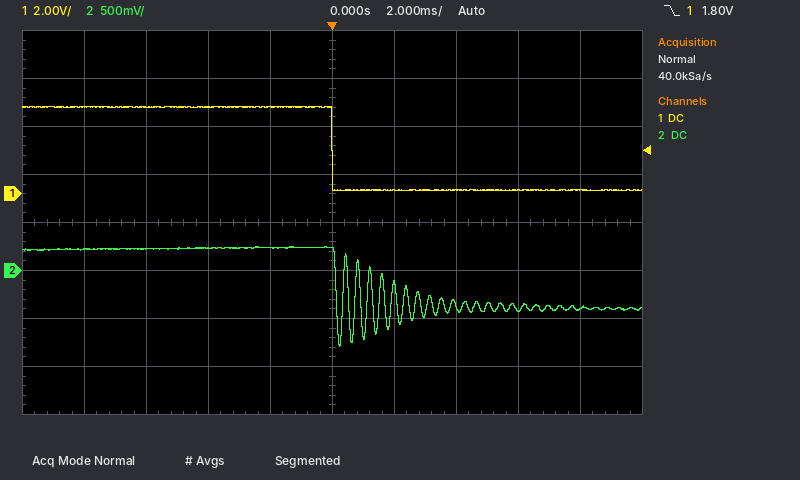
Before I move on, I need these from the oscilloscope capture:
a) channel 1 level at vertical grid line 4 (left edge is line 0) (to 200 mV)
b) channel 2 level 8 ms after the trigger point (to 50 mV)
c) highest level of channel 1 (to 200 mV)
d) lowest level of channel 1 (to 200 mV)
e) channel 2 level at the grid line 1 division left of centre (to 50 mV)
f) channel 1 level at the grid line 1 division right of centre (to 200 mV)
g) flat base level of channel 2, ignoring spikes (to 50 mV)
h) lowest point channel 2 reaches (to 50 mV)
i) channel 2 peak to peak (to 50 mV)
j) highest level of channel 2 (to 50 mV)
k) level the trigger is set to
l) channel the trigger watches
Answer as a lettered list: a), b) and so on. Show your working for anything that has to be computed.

a) 3.6 V
b) -400 mV
c) 3.6 V
d) 200 mV
e) 250 mV
f) 200 mV
g) -400 mV
h) -800 mV
i) 250 mV − (-800 mV) = 1.05 V
j) 250 mV
k) 1.80 V
l) channel 1
